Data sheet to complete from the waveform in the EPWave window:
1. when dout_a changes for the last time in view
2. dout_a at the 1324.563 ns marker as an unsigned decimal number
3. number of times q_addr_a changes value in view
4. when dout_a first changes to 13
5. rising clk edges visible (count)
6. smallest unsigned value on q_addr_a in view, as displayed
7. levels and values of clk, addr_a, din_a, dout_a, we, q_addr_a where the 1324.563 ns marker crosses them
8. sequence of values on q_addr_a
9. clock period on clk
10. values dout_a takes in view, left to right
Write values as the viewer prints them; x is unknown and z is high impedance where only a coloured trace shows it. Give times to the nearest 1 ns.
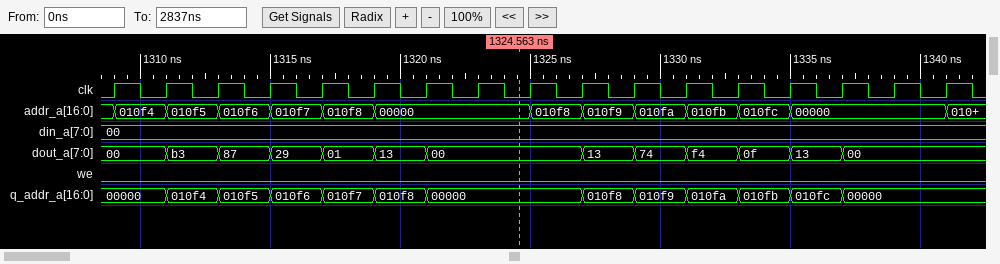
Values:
1337 ns
0
12
1319 ns
17
00000
clk=0, addr_a=00000, din_a=00, dout_a=00, we=0, q_addr_a=00000
00000, 010f4, 010f5, 010f6, 010f7, 010f8, 00000, 010f8, 010f9, 010fa, 010fb, 010fc, 00000
2 ns
00, b3, 87, 29, 01, 13, 00, 13, 74, f4, 0f, 13, 00
